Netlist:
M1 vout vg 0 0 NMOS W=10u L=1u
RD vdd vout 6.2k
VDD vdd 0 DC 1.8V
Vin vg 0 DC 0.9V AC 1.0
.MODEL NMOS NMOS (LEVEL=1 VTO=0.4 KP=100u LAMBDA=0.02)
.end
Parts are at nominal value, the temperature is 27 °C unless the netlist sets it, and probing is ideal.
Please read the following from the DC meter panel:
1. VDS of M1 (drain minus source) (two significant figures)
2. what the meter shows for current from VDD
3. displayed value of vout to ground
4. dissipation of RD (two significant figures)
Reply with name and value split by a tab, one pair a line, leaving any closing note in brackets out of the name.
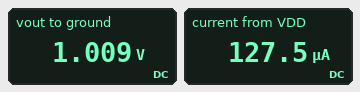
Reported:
VDS of M1 (drain minus source)	1.0 V
what the meter shows for current from VDD	127.5 µA
displayed value of vout to ground	1.009 V
dissipation of RD	100 µW
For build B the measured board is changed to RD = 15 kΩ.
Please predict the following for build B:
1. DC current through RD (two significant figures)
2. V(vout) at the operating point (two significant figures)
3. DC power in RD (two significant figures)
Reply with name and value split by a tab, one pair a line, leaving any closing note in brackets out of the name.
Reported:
DC current through RD	100 µA
V(vout) at the operating point	280 mV
DC power in RD	150 µW
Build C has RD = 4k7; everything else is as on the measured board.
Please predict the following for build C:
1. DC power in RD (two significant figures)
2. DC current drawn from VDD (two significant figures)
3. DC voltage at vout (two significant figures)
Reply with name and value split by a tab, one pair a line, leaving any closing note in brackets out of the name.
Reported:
DC power in RD	77 µW
DC current drawn from VDD	130 µA
DC voltage at vout	1.2 V
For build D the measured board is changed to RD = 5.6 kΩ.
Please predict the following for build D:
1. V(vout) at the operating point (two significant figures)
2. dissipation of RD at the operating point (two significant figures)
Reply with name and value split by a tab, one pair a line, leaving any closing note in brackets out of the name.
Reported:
V(vout) at the operating point	1.1 V
dissipation of RD at the operating point	91 µW
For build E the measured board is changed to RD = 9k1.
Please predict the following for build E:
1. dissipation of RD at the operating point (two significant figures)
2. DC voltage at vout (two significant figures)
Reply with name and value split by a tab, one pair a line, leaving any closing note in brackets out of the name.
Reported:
dissipation of RD at the operating point	150 µW
DC voltage at vout	650 mV
